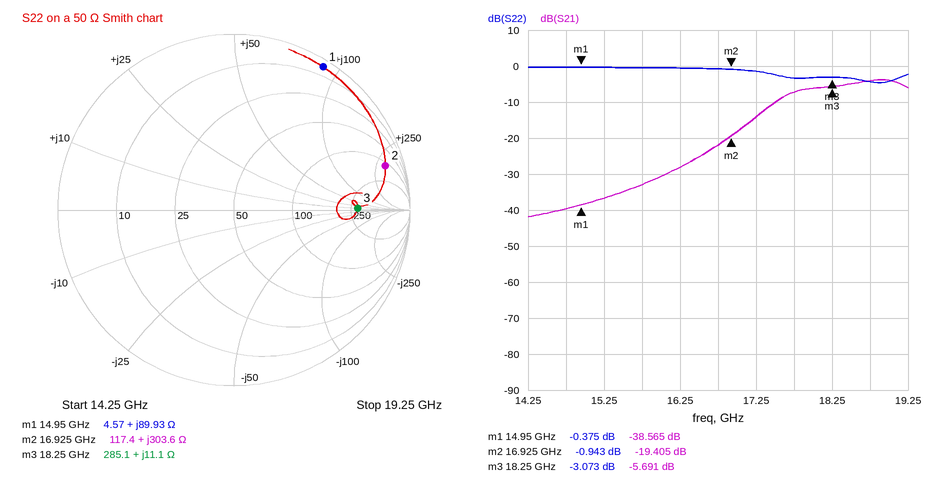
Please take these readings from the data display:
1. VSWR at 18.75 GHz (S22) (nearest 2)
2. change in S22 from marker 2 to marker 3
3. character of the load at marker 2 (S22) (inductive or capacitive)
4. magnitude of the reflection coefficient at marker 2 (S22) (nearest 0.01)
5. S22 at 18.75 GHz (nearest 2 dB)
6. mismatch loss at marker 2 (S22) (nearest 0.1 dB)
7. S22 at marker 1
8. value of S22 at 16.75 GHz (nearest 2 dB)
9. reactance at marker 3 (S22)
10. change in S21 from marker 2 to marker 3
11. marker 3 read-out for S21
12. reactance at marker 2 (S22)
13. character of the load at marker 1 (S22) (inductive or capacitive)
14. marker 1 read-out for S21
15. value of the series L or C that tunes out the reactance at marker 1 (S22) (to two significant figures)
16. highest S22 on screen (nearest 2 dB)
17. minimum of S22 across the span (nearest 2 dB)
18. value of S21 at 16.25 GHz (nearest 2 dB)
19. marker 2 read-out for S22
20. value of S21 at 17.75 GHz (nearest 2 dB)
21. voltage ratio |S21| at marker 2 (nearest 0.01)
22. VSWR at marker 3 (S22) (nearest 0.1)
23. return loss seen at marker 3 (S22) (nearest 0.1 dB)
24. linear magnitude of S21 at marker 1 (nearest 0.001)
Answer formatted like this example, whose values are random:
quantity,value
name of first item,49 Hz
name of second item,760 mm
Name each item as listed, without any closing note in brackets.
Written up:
quantity,value
VSWR at 18.75 GHz (S22),4
change in S22 from marker 2 to marker 3,-2.130 dB
character of the load at marker 2 (S22),inductive
magnitude of the reflection coefficient at marker 2 (S22),0.90
S22 at 18.75 GHz,-4 dB
mismatch loss at marker 2 (S22),7.1 dB
S22 at marker 1,-0.375 dB
value of S22 at 16.75 GHz,0 dB
reactance at marker 3,+11.1 Ω
change in S21 from marker 2 to marker 3,13.714 dB
marker 3 read-out for S21,-5.691 dB
reactance at marker 2,+303.6 Ω
character of the load at marker 1 (S22),inductive
marker 1 read-out for S21,-38.565 dB
value of the series L or C that tunes out the reactance at marker 1 (S22),120 fF
highest S22 on screen,0 dB
minimum of S22 across the span,-4 dB
value of S21 at 16.25 GHz,-28 dB
marker 2 read-out for S22,-0.943 dB
value of S21 at 17.75 GHz,-8 dB
voltage ratio |S21| at marker 2,0.11
VSWR at marker 3 (S22),5.7
return loss seen at marker 3 (S22),3.1 dB
linear magnitude of S21 at marker 1,0.012
